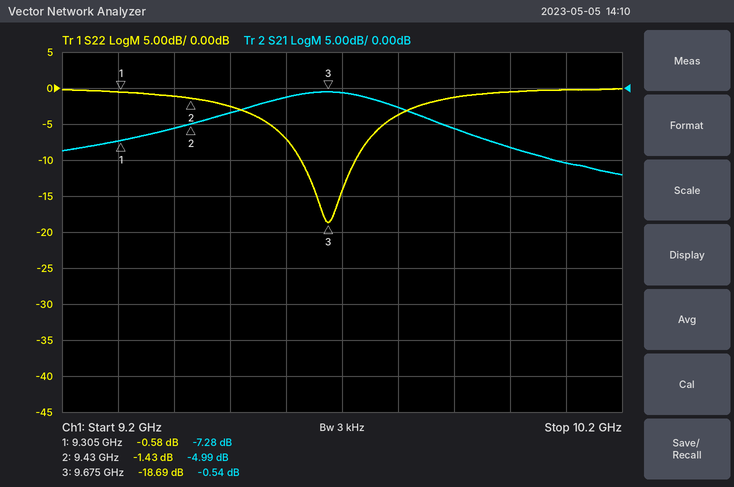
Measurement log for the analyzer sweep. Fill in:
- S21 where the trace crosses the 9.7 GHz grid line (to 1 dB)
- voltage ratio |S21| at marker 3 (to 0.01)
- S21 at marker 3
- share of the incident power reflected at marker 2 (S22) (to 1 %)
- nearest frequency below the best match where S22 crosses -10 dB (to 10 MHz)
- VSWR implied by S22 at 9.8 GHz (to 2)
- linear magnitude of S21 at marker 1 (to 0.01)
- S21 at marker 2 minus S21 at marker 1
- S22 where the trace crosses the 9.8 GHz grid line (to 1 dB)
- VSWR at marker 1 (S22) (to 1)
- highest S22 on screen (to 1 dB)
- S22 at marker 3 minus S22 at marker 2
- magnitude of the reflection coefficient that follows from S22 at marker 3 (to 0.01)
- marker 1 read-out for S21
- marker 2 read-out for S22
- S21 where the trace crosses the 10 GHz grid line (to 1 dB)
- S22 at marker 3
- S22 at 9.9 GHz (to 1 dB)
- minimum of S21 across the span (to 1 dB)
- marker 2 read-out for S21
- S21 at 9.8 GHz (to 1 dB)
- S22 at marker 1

-1 dB
0.94
-0.54 dB
72 %
9.63 GHz
4
0.43
2.29 dB
-4 dB
30
0 dB
-17.26 dB
0.12
-7.28 dB
-1.43 dB
-8 dB
-18.69 dB
-1 dB
-12 dB
-4.99 dB
-3 dB
-0.58 dB
